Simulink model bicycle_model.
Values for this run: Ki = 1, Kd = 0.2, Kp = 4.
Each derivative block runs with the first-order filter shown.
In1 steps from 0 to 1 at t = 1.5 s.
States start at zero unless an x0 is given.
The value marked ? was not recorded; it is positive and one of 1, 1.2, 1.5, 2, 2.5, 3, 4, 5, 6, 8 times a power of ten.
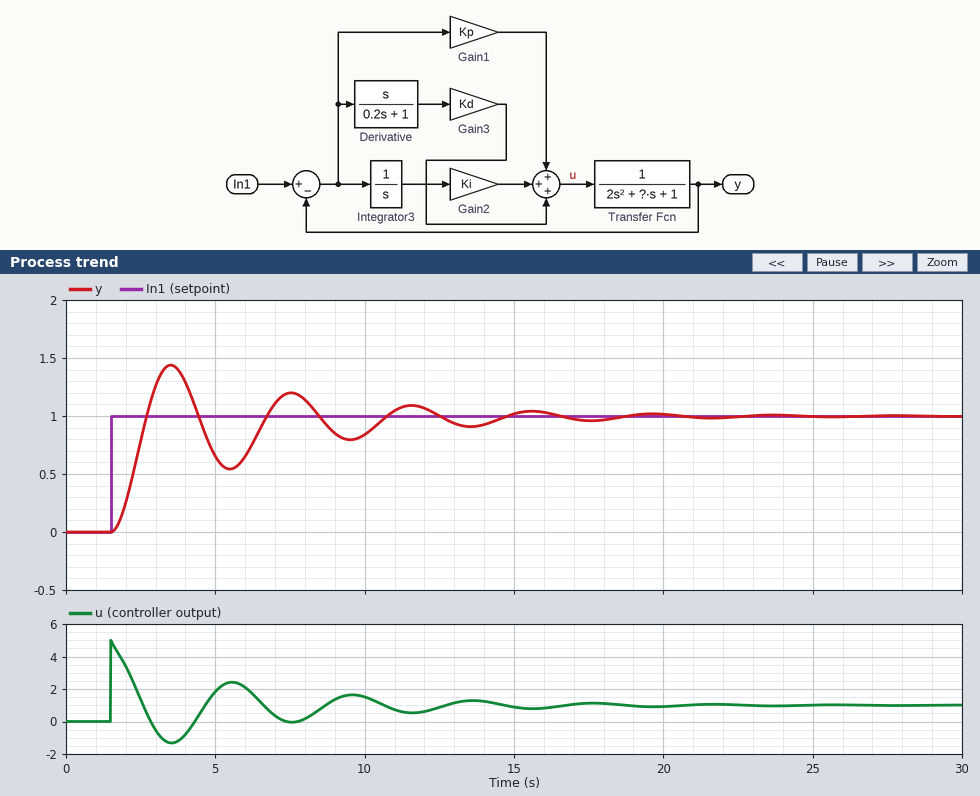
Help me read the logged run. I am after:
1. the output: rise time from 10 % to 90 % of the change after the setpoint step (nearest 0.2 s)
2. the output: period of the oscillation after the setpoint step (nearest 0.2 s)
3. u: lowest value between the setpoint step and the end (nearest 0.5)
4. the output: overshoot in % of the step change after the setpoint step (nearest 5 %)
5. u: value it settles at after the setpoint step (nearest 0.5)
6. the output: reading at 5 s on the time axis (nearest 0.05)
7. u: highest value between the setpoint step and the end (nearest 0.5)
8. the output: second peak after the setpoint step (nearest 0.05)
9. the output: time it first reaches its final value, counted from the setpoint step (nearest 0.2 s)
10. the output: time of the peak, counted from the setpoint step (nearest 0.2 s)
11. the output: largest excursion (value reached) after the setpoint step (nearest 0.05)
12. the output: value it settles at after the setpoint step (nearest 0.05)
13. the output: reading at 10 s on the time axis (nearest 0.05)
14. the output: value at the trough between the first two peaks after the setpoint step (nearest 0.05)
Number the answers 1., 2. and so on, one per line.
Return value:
1. 0.8 s
2. 4.0 s
3. -1.5
4. 45 %
5. 1.0
6. 0.65
7. 5.0
8. 1.20
9. 1.2 s
10. 2.0 s
11. 1.45
12. 1.00
13. 0.85
14. 0.55
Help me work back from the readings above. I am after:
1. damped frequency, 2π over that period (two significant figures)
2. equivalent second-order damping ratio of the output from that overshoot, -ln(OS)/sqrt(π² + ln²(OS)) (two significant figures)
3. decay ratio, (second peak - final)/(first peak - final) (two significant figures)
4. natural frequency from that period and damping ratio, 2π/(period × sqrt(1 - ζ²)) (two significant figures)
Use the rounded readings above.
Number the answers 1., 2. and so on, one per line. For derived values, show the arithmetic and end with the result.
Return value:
1. 2π / 4 = 1.6 rad/s
2. ln(0.45) = -0.799; 0.799 / sqrt(9.870 + 0.638) = 0.25
3. (1.2 - 1) / (1.45 - 1) = 0.44
4. 2π / (4 × sqrt(1 - 0.25²)) = 1.6 rad/s
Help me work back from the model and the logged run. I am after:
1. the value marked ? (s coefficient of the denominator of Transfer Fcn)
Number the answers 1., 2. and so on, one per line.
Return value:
1. 1
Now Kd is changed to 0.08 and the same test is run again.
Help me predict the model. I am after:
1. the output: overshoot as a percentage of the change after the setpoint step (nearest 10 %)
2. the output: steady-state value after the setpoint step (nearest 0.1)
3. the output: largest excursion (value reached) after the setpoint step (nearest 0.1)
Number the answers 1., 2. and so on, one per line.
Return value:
1. 50 %
2. 1.0
3. 1.5
